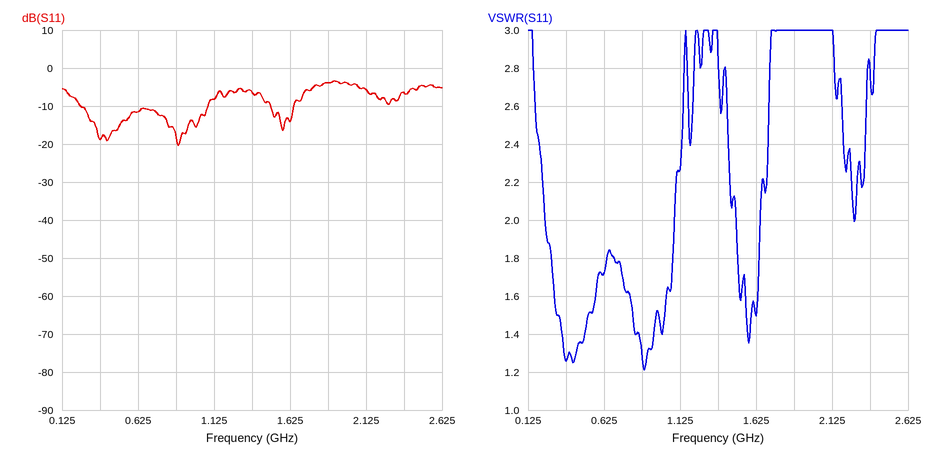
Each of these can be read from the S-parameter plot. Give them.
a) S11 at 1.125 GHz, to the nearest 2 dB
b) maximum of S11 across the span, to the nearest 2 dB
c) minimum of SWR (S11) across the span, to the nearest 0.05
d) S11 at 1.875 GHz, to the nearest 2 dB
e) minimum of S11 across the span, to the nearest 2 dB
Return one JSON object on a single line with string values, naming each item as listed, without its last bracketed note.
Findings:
{"S11 at 1.125 GHz, to the nearest 2 dB": "-8 dB", "maximum of S11 across the span, to the nearest 2 dB": "-4 dB", "minimum of SWR (S11) across the span, to the nearest 0.05": "1.20", "S11 at 1.875 GHz, to the nearest 2 dB": "-4 dB", "minimum of S11 across the span, to the nearest 2 dB": "-20 dB"}
